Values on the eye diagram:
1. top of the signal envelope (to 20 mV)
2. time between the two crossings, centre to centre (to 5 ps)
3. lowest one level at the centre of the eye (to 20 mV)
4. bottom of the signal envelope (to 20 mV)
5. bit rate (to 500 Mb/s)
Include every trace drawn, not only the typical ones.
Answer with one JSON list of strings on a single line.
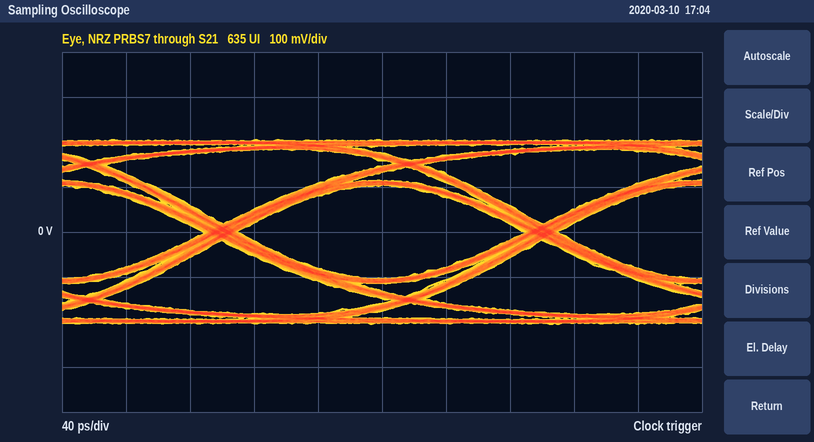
["200 mV", "200 ps", "100 mV", "-200 mV", "5.0 Gb/s"]
